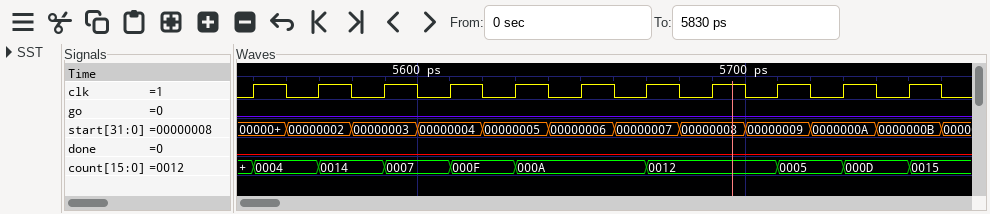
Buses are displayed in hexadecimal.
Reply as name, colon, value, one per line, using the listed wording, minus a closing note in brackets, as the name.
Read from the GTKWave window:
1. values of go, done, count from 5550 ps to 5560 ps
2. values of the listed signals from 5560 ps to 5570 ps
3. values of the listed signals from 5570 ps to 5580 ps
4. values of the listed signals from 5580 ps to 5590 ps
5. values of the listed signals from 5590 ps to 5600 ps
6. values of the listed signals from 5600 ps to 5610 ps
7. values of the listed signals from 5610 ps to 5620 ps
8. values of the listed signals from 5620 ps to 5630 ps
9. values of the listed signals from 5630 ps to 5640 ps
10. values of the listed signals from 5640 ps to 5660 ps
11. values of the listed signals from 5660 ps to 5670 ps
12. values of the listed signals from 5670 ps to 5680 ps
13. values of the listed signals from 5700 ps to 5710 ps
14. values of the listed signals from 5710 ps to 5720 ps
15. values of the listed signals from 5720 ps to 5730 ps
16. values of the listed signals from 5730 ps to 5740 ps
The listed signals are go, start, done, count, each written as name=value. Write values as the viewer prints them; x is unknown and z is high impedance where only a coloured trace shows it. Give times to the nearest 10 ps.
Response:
values of go, done, count from 5550 ps to 5560 ps: go=0, done=0, count=0004
values of the listed signals from 5560 ps to 5570 ps: go=0, start=00000002, done=0, count=0004
values of the listed signals from 5570 ps to 5580 ps: go=0, start=00000002, done=0, count=0014
values of the listed signals from 5580 ps to 5590 ps: go=0, start=00000003, done=0, count=0014
values of the listed signals from 5590 ps to 5600 ps: go=0, start=00000003, done=0, count=0007
values of the listed signals from 5600 ps to 5610 ps: go=0, start=00000004, done=0, count=0007
values of the listed signals from 5610 ps to 5620 ps: go=0, start=00000004, done=0, count=000F
values of the listed signals from 5620 ps to 5630 ps: go=0, start=00000005, done=0, count=000F
values of the listed signals from 5630 ps to 5640 ps: go=0, start=00000005, done=0, count=000A
values of the listed signals from 5640 ps to 5660 ps: go=0, start=00000006, done=0, count=000A
values of the listed signals from 5660 ps to 5670 ps: go=0, start=00000007, done=0, count=000A
values of the listed signals from 5670 ps to 5680 ps: go=0, start=00000007, done=0, count=0012
values of the listed signals from 5700 ps to 5710 ps: go=0, start=00000009, done=0, count=0012
values of the listed signals from 5710 ps to 5720 ps: go=0, start=00000009, done=0, count=0005
values of the listed signals from 5720 ps to 5730 ps: go=0, start=0000000A, done=0, count=0005
values of the listed signals from 5730 ps to 5740 ps: go=0, start=0000000A, done=0, count=000D
